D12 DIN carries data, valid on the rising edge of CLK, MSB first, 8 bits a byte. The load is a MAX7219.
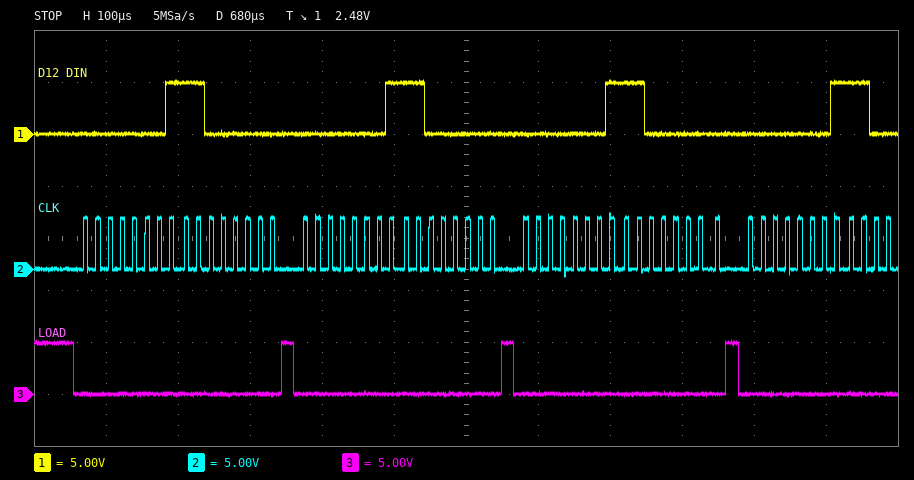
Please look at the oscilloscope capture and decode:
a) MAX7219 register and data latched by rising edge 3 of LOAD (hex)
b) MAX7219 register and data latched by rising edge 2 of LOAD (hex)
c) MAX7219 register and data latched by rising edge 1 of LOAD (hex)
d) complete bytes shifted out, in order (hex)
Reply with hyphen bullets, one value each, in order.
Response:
- register 0x1, data 0xC0
- register 0x1, data 0xC0
- register 0x1, data 0xC0
- 0x01 0xC0 0x01 0xC0 0x01 0xC0 0x01
